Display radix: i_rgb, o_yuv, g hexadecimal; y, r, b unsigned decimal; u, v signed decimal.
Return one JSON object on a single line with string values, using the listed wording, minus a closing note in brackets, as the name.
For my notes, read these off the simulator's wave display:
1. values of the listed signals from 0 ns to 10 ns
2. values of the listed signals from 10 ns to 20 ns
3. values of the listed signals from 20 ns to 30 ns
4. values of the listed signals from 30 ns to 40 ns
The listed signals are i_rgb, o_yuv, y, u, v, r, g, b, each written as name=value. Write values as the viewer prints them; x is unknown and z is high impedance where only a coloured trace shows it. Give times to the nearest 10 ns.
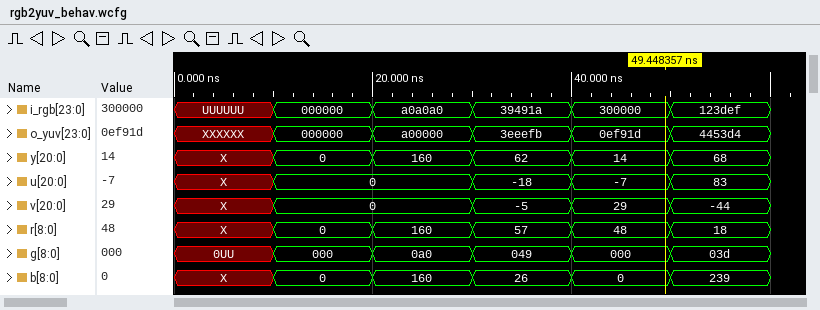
{"values of the listed signals from 0 ns to 10 ns": "i_rgb=UUUUUU, o_yuv=XXXXXX, y=X, u=X, v=X, r=X, g=0UU, b=X", "values of the listed signals from 10 ns to 20 ns": "i_rgb=000000, o_yuv=000000, y=0, u=0, v=0, r=0, g=000, b=0", "values of the listed signals from 20 ns to 30 ns": "i_rgb=a0a0a0, o_yuv=a00000, y=160, u=0, v=0, r=160, g=0a0, b=160", "values of the listed signals from 30 ns to 40 ns": "i_rgb=39491a, o_yuv=3eeefb, y=62, u=-18, v=-5, r=57, g=049, b=26"}
